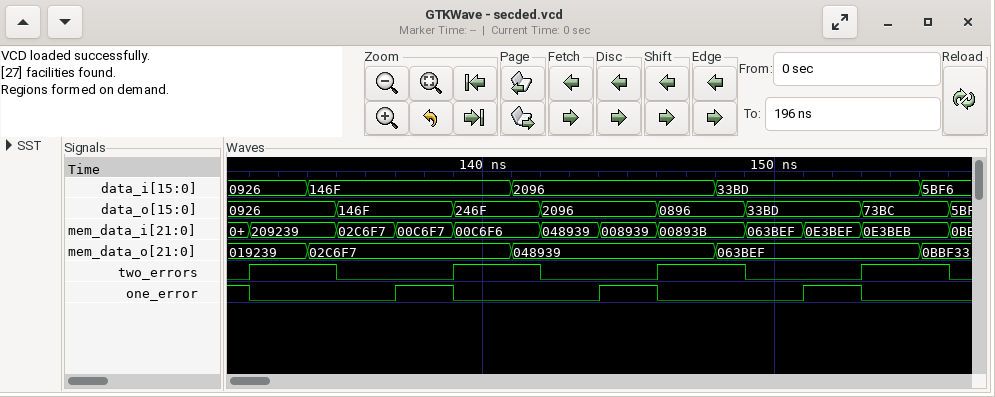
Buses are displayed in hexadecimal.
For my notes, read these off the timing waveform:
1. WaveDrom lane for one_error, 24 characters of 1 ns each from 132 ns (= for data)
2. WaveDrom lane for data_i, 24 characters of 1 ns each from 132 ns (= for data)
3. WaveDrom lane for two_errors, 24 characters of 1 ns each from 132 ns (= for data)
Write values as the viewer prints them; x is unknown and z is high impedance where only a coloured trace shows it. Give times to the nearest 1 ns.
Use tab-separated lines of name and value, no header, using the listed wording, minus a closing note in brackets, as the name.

WaveDrom lane for one_error, 24 characters of 1 ns each from 132 ns	{name: 'one_error', wave: '0....1.0....1.0....1.0..'}
WaveDrom lane for data_i, 24 characters of 1 ns each from 132 ns	{name: 'data_i', wave: '=.=......=......=......=', data: '0926 146F 2096 33BD 5BF6'}
WaveDrom lane for two_errors, 24 characters of 1 ns each from 132 ns	{name: 'two_errors', wave: '1..0...1..0...1..0...1..'}
